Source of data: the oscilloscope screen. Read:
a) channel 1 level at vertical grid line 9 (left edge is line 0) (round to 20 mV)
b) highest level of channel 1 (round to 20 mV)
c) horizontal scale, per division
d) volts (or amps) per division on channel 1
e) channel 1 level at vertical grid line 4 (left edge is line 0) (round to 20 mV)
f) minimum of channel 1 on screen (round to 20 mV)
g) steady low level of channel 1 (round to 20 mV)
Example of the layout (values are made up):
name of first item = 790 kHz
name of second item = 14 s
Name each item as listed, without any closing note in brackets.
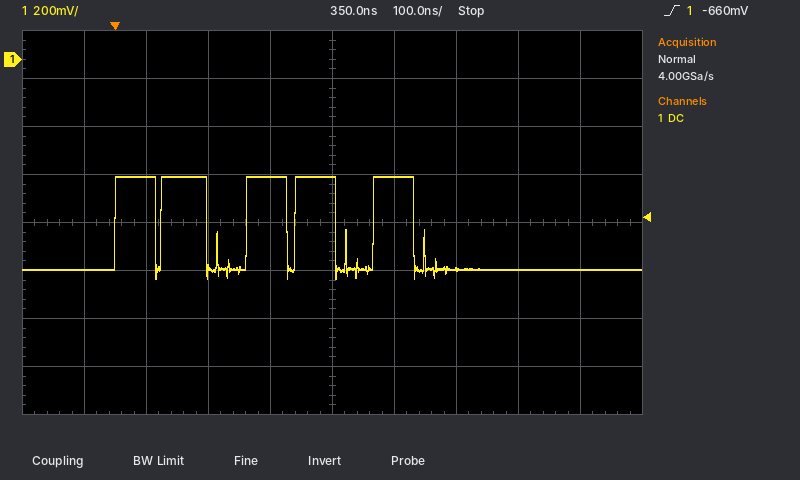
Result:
channel 1 level at vertical grid line 9 (left edge is line 0) = -880 mV
highest level of channel 1 = -480 mV
horizontal scale, per division = 100 ns
volts (or amps) per division on channel 1 = 200 mV
channel 1 level at vertical grid line 4 (left edge is line 0) = -480 mV
minimum of channel 1 on screen = -920 mV
steady low level of channel 1 = -880 mV
